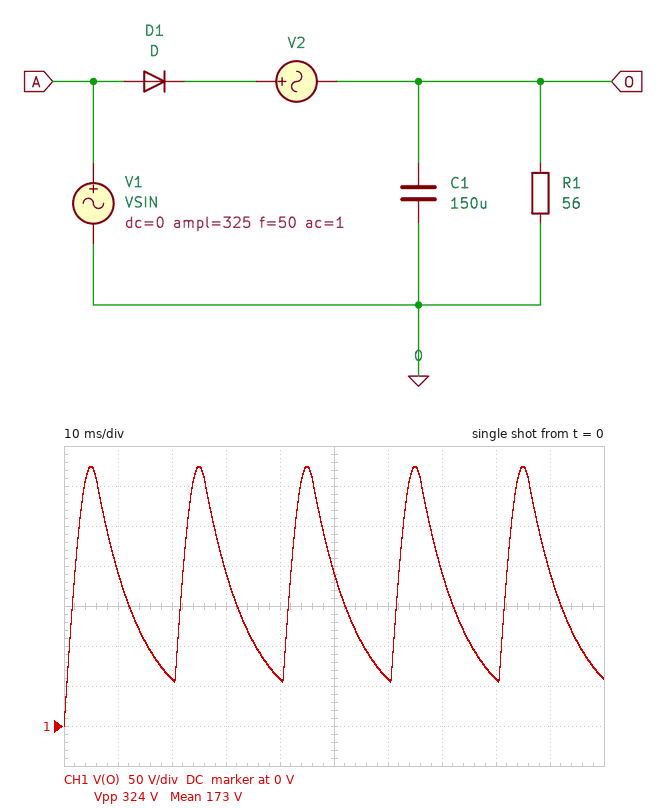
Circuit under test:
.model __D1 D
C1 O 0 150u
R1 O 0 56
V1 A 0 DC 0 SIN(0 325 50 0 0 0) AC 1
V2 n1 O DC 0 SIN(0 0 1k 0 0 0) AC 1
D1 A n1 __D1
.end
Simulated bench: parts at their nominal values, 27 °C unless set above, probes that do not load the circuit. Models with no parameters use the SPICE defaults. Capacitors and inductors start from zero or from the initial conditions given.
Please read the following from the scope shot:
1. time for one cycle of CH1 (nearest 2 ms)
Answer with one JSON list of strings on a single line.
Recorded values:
["20 ms"]
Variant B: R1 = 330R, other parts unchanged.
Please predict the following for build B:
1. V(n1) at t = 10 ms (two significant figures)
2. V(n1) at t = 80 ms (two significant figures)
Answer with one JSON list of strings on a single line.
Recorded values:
["290 V", "240 V"]
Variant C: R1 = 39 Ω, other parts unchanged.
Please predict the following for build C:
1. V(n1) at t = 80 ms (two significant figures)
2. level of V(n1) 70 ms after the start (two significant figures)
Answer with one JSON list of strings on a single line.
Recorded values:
["29 V", "160 V"]
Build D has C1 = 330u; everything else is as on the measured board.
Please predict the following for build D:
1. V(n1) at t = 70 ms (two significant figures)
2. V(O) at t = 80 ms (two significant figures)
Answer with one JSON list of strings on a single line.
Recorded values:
["250 V", "150 V"]
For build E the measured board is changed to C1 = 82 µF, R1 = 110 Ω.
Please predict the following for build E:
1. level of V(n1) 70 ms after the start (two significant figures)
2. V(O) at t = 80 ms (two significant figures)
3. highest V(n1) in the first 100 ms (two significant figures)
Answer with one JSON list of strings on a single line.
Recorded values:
["200 V", "65 V", "320 V"]
